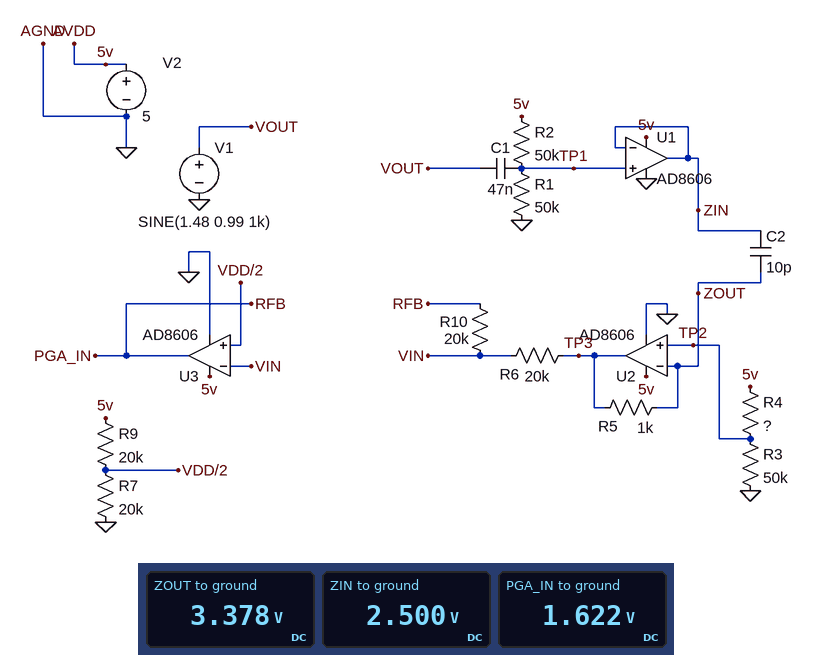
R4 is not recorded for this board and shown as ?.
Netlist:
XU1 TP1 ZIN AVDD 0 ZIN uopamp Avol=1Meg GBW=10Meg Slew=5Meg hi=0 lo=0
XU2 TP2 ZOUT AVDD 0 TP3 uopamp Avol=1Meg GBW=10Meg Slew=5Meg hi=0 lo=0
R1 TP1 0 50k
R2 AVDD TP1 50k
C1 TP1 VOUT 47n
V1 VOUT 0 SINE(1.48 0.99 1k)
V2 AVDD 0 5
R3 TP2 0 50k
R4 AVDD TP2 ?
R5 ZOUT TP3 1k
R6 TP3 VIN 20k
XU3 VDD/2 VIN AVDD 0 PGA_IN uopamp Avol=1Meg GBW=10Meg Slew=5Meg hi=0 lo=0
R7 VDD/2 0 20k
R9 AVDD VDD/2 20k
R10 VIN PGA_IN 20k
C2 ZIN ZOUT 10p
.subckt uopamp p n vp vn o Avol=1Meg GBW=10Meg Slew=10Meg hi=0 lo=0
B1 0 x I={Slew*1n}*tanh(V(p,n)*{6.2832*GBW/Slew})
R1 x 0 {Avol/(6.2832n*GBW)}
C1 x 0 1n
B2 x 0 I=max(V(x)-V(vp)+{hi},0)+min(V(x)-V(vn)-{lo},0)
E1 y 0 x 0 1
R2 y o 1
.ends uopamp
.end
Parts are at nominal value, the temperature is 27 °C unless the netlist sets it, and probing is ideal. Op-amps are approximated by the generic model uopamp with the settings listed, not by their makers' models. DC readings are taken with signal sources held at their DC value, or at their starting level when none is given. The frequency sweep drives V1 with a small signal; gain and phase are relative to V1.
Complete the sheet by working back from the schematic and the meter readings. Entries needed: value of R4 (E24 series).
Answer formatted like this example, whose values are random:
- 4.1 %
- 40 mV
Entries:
- 24 kΩ
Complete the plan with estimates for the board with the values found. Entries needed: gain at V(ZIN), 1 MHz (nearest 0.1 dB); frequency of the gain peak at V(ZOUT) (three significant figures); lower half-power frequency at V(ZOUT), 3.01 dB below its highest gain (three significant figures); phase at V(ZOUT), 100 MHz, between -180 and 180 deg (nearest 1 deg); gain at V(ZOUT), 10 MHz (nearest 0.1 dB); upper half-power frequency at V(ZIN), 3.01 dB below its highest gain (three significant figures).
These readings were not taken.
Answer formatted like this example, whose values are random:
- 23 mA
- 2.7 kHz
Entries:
- 0 dB
- 14.4 MHz
- 8.77 MHz
- -75 deg
- -7.6 dB
- 10.0 MHz
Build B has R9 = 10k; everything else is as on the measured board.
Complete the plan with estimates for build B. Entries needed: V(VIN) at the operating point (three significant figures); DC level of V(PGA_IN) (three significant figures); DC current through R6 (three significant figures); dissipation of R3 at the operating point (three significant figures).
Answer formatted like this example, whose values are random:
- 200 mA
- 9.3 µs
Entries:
- 3.33 V
- 3.29 V
- 2.25 µA
- 228 µW
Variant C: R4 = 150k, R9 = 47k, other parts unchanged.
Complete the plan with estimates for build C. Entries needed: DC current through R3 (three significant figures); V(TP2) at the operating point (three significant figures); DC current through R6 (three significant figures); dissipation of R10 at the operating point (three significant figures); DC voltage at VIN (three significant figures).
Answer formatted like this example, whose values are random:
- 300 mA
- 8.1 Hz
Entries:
- 25.0 µA
- 1.25 V
- 12.1 µA
- 2.94 µW
- 1.49 V
